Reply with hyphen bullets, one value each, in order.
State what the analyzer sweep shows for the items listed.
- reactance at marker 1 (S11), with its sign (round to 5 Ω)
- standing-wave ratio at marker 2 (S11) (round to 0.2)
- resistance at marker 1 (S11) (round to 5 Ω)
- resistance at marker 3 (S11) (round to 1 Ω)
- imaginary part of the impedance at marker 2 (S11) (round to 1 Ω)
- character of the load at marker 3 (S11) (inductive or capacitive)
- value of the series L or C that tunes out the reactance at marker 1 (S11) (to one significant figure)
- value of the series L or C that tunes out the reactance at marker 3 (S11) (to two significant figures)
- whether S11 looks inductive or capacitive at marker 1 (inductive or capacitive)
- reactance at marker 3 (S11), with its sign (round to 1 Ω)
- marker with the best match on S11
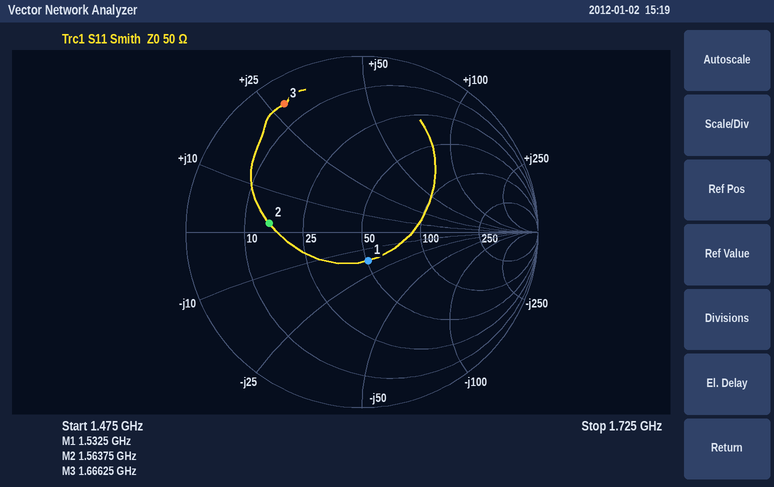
- -15 Ω
- 3.2
- 50 Ω
- 5 Ω
- +2 Ω
- inductive
- 2 nH
- 3.4 pF
- capacitive
- +28 Ω
- marker 1
